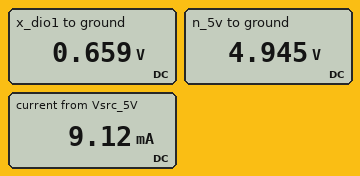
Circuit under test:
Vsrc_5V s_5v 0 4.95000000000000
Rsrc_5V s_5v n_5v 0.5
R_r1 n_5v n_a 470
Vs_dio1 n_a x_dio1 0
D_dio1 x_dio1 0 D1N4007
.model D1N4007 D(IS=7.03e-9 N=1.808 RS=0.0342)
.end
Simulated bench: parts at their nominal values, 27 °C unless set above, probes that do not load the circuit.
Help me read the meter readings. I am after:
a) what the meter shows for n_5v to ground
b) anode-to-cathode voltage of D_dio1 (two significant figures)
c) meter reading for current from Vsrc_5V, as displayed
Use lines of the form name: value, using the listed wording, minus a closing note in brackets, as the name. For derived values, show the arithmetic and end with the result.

what the meter shows for n_5v to ground: 4.945 V
anode-to-cathode voltage of D_dio1: 659 mV = 660 mV
meter reading for current from Vsrc_5V, as displayed: 9.12 mA
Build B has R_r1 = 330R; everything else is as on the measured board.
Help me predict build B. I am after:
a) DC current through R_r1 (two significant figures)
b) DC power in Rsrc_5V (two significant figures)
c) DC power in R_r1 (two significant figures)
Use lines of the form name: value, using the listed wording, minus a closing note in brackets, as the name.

DC current through R_r1: 13 mA
DC power in Rsrc_5V: 84 µW
DC power in R_r1: 55 mW
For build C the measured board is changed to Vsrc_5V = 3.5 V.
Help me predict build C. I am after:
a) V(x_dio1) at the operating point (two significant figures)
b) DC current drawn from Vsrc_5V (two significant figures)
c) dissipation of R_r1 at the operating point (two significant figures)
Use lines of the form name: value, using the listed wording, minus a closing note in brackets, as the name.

V(x_dio1) at the operating point: 640 mV
DC current drawn from Vsrc_5V: 6.1 mA
dissipation of R_r1 at the operating point: 17 mW
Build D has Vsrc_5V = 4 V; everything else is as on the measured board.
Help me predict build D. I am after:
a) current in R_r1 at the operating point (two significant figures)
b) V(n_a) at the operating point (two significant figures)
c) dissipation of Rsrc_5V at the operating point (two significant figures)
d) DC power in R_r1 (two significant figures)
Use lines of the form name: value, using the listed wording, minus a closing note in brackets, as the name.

current in R_r1 at the operating point: 7.1 mA
V(n_a) at the operating point: 650 mV
dissipation of Rsrc_5V at the operating point: 25 µW
DC power in R_r1: 24 mW
